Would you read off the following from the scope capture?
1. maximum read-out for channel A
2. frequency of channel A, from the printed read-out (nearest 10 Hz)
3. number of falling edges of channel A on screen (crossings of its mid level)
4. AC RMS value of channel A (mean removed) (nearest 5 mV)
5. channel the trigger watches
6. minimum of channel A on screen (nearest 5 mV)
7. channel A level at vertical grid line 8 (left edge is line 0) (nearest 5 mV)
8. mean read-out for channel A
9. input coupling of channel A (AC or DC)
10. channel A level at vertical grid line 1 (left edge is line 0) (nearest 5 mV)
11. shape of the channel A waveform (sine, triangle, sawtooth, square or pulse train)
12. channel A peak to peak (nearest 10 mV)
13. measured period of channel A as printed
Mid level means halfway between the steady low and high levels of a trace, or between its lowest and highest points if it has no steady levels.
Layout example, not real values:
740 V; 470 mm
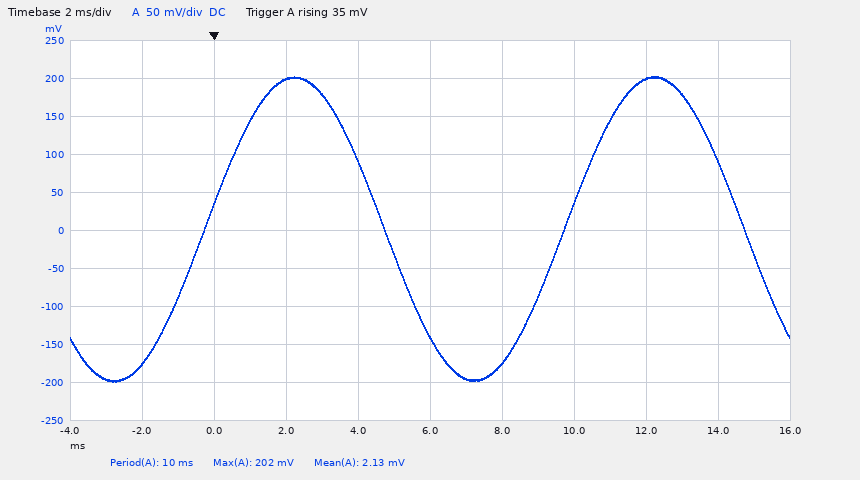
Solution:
202 mV; 100 Hz; 2; 140 mV; channel A; -200 mV; 200 mV; 2.13 mV; DC; -175 mV; sine; 400 mV; 10 ms
